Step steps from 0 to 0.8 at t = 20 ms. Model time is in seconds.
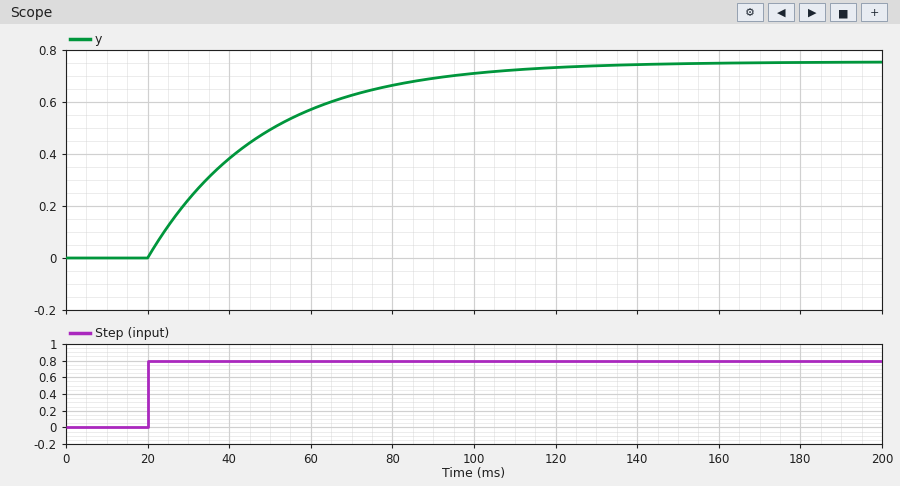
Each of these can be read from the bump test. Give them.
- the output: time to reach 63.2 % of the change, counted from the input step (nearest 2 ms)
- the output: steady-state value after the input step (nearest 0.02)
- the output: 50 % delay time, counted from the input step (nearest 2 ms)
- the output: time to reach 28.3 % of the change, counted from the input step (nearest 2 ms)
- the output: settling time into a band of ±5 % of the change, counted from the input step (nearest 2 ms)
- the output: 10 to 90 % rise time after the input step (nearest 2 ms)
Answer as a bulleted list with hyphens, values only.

- 28 ms
- 0.76
- 20 ms
- 10 ms
- 84 ms
- 62 ms
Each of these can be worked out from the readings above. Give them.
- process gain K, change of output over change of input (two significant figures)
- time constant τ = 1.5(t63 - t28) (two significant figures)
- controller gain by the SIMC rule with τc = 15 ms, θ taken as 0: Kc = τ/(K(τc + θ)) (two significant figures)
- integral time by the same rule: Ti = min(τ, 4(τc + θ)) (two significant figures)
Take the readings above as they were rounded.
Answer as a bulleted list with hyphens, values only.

- 0.95
- 27 ms
- 1.9
- 27 ms
